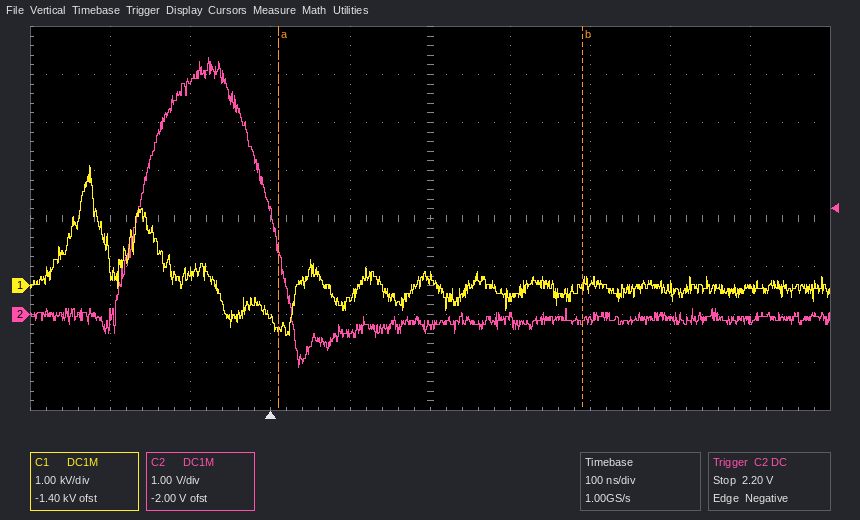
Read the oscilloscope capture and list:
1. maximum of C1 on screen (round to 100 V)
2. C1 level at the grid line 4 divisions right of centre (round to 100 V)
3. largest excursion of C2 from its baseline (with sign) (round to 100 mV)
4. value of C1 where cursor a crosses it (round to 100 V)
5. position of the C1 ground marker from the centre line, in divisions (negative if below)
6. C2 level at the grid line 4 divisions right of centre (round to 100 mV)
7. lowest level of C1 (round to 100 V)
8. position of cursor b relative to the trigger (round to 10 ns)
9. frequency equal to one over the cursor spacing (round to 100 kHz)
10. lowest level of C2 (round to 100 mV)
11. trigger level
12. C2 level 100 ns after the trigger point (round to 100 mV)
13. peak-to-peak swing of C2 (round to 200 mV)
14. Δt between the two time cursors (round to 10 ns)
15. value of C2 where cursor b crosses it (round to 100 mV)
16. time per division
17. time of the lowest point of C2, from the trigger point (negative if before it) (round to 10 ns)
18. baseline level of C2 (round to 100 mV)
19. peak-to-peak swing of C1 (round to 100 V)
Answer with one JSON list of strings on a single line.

["2.5 kV", "-100 V", "+5.4 V", "-900 V", "-1.4 div", "-100 mV", "-1.0 kV", "+390 ns", "2.6 MHz", "-1.1 V", "2.20 V", "-400 mV", "6.4 V", "380 ns", "-100 mV", "100 ns", "+40 ns", "-100 mV", "3.5 kV"]
